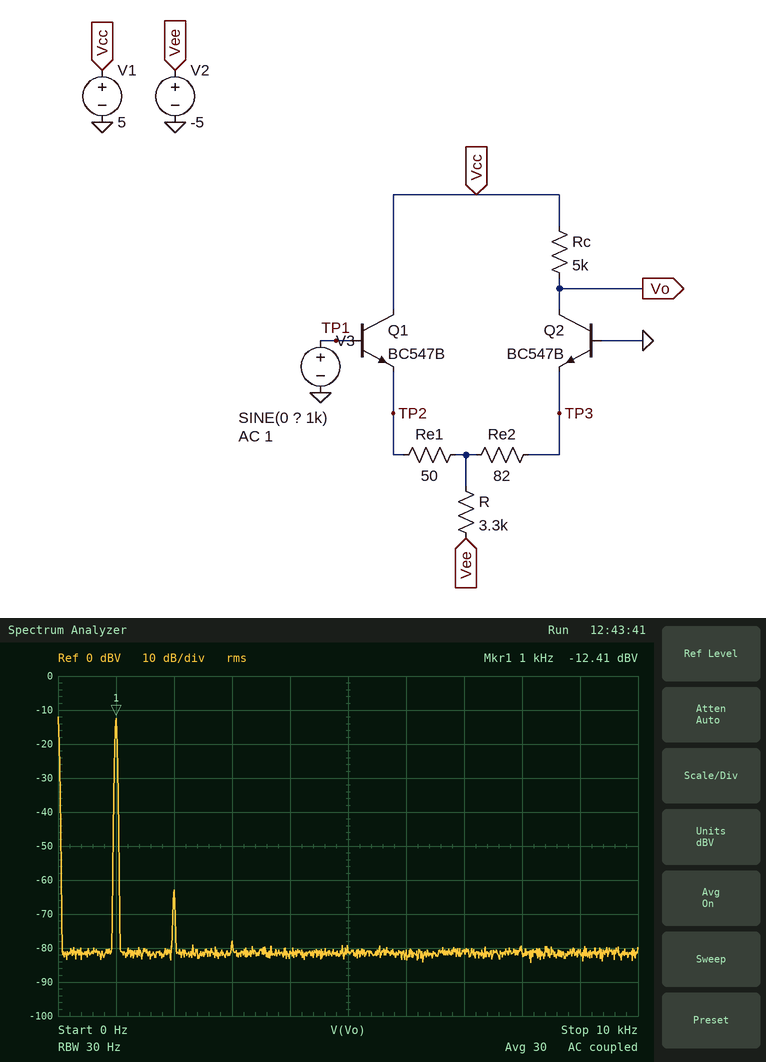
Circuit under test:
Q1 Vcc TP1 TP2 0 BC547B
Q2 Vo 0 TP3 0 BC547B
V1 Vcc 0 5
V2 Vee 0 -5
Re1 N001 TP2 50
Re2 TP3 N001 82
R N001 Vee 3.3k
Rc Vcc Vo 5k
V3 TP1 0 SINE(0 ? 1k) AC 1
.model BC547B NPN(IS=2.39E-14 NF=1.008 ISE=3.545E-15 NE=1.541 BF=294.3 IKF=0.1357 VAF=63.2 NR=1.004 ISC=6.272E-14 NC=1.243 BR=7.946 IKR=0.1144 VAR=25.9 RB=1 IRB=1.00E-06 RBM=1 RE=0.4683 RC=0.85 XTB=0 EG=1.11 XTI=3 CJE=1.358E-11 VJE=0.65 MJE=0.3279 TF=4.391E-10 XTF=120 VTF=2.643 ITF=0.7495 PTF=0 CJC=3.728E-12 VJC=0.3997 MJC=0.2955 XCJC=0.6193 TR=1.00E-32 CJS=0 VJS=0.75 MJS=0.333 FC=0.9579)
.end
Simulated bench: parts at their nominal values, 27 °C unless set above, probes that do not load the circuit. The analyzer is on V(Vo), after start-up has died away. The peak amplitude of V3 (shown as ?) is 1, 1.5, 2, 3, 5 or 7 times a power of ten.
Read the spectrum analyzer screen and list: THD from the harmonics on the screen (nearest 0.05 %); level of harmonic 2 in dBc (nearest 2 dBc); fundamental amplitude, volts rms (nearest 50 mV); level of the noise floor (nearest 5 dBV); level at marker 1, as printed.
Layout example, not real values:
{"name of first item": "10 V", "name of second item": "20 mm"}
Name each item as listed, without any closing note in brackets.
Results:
{"THD from the harmonics on the screen": "0.30 %", "level of harmonic 2 in dBc": "-50 dBc", "fundamental amplitude, volts rms": "250 mV", "level of the noise floor": "-80 dBV", "level at marker 1, as printed": "-12.41 dBV"}
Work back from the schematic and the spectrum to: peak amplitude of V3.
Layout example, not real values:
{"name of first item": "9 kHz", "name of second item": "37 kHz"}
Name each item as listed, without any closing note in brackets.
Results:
{"peak amplitude of V3": "15 mV"}
